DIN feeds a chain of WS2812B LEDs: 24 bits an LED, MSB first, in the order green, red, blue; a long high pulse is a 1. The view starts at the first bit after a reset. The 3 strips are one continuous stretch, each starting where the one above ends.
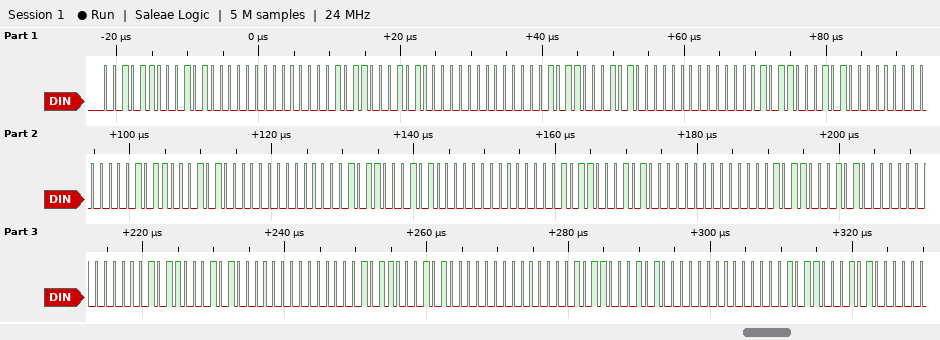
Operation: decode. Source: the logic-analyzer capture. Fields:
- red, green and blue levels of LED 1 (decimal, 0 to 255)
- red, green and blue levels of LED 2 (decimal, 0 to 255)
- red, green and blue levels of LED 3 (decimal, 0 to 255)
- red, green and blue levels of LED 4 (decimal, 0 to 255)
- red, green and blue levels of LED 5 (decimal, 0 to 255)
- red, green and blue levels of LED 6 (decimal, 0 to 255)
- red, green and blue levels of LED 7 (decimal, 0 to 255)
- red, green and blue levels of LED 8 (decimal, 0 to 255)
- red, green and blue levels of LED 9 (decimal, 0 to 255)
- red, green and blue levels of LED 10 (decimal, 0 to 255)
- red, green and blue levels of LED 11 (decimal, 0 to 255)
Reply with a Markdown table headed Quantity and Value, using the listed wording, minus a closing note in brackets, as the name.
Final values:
| Quantity | Value |
|---|---|
| red, green and blue levels of LED 1 | 80, 44, 0 |
| red, green and blue levels of LED 2 | 80, 44, 0 |
| red, green and blue levels of LED 3 | 80, 44, 0 |
| red, green and blue levels of LED 4 | 80, 44, 0 |
| red, green and blue levels of LED 5 | 80, 44, 0 |
| red, green and blue levels of LED 6 | 80, 44, 0 |
| red, green and blue levels of LED 7 | 80, 44, 0 |
| red, green and blue levels of LED 8 | 80, 44, 0 |
| red, green and blue levels of LED 9 | 80, 44, 0 |
| red, green and blue levels of LED 10 | 80, 44, 0 |
| red, green and blue levels of LED 11 | 80, 44, 0 |
